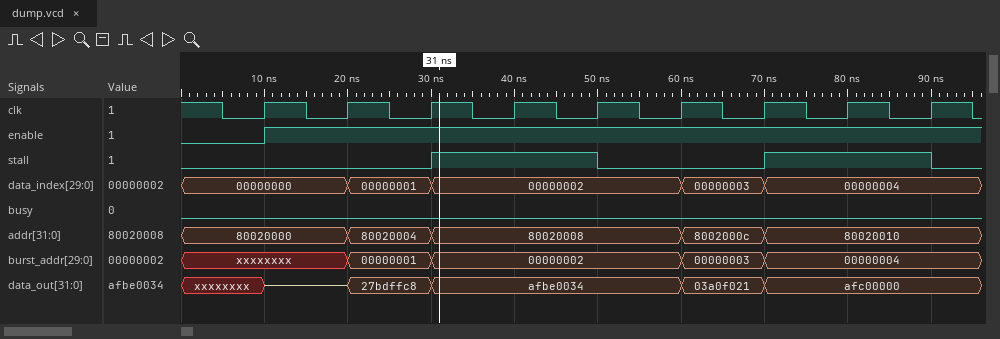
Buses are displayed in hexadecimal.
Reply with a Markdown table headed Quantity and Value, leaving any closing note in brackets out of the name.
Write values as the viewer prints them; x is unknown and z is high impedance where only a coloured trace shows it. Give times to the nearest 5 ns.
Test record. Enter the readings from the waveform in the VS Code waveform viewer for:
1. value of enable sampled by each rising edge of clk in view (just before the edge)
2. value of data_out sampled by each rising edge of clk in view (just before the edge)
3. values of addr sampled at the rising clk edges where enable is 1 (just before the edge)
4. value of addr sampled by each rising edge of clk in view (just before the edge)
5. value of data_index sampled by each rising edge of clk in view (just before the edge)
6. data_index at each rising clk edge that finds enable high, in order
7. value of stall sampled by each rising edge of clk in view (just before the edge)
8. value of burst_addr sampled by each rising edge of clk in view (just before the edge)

| Quantity | Value |
|---|---|
| value of enable sampled by each rising edge of clk in view | 0 1 1 1 1 1 1 1 1 |
| value of data_out sampled by each rising edge of clk in view | xxxxxxxx, z, 27bdffc8, afbe0034, afbe0034, afbe0034, 03a0f021, afc00000, afc00000 |
| values of addr sampled at the rising clk edges where enable is 1 | 80020000, 80020004, 80020008, 80020008, 80020008, 8002000c, 80020010, 80020010 |
| value of addr sampled by each rising edge of clk in view | 80020000, 80020000, 80020004, 80020008, 80020008, 80020008, 8002000c, 80020010, 80020010 |
| value of data_index sampled by each rising edge of clk in view | 00000000, 00000000, 00000001, 00000002, 00000002, 00000002, 00000003, 00000004, 00000004 |
| data_index at each rising clk edge that finds enable high, in order | 00000000, 00000001, 00000002, 00000002, 00000002, 00000003, 00000004, 00000004 |
| value of stall sampled by each rising edge of clk in view | 0 0 0 1 1 0 0 1 1 |
| value of burst_addr sampled by each rising edge of clk in view | xxxxxxxx, xxxxxxxx, 00000001, 00000002, 00000002, 00000002, 00000003, 00000004, 00000004 |
